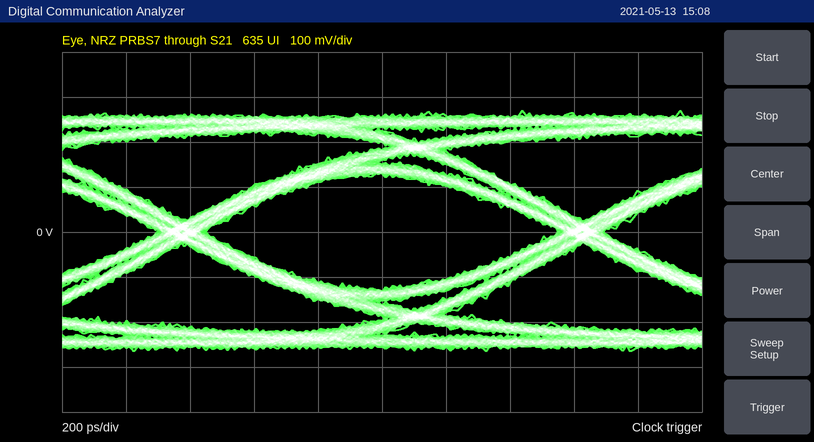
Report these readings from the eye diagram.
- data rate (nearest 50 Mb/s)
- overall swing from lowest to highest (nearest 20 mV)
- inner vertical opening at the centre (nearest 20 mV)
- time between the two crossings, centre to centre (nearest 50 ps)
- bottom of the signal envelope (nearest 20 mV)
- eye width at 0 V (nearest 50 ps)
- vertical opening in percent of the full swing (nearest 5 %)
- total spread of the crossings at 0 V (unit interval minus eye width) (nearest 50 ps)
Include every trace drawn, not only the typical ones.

800 Mb/s
540 mV
260 mV
1.25 ns
-260 mV
1.10 ns
50 %
150 ps
